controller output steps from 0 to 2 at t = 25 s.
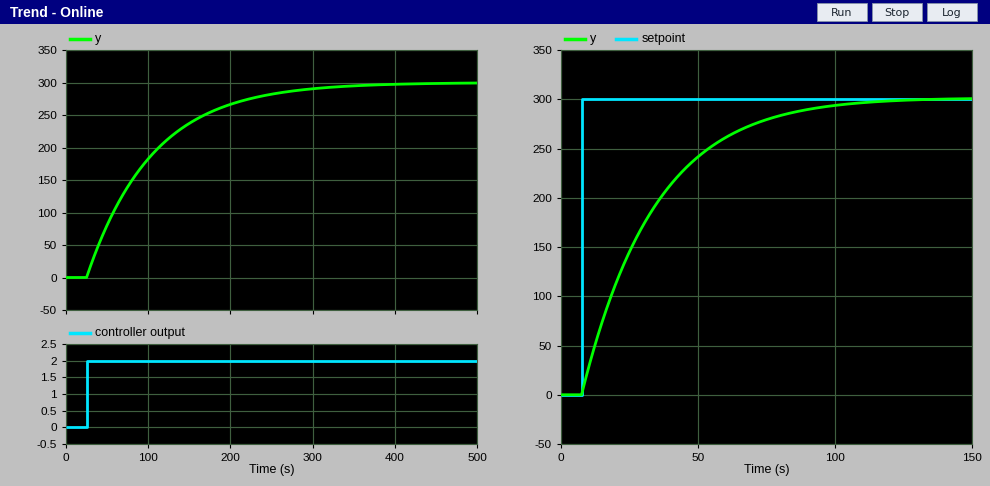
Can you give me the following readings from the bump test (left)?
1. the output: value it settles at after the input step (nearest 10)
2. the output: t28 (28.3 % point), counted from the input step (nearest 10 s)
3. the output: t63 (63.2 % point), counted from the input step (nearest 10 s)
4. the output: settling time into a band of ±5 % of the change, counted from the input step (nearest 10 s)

300
30 s
80 s
240 s
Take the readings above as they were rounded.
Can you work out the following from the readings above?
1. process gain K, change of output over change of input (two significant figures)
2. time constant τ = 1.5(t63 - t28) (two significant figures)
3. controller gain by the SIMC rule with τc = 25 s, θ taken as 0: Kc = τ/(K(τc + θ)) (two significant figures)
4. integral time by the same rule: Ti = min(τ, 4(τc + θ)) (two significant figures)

150
75 s
0.020
75 s
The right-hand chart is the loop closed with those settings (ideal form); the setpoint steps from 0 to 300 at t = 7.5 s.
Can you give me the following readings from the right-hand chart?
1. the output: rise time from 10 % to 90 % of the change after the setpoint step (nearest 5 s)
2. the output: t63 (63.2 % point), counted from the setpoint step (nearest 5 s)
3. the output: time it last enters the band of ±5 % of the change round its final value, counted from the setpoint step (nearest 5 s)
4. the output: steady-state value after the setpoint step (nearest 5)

55 s
25 s
75 s
300
